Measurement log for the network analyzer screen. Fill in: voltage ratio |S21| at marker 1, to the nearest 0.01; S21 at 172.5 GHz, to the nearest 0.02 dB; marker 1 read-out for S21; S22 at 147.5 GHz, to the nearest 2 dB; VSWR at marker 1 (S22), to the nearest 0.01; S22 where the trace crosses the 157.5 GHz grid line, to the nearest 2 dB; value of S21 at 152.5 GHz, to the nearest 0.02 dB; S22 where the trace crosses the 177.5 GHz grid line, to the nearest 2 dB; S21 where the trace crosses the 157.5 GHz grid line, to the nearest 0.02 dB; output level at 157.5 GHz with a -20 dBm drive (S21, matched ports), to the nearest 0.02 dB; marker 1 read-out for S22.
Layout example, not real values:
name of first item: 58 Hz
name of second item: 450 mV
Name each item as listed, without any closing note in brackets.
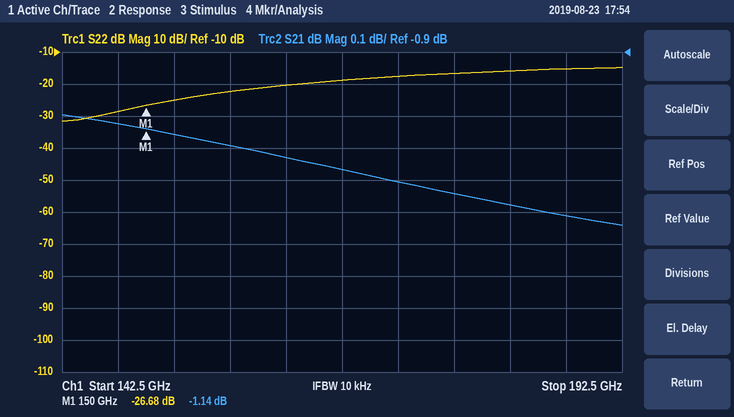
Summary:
voltage ratio |S21| at marker 1, to the nearest 0.01: 0.88
S21 at 172.5 GHz, to the nearest 0.02 dB: -1.30 dB
marker 1 read-out for S21: -1.14 dB
S22 at 147.5 GHz, to the nearest 2 dB: -28 dB
VSWR at marker 1 (S22), to the nearest 0.01: 1.10
S22 where the trace crosses the 157.5 GHz grid line, to the nearest 2 dB: -22 dB
value of S21 at 152.5 GHz, to the nearest 0.02 dB: -1.16 dB
S22 where the trace crosses the 177.5 GHz grid line, to the nearest 2 dB: -16 dB
S21 where the trace crosses the 157.5 GHz grid line, to the nearest 0.02 dB: -1.20 dB
output level at 157.5 GHz with a -20 dBm drive (S21, matched ports), to the nearest 0.02 dB: -21.20 dBm
marker 1 read-out for S22: -26.68 dB
